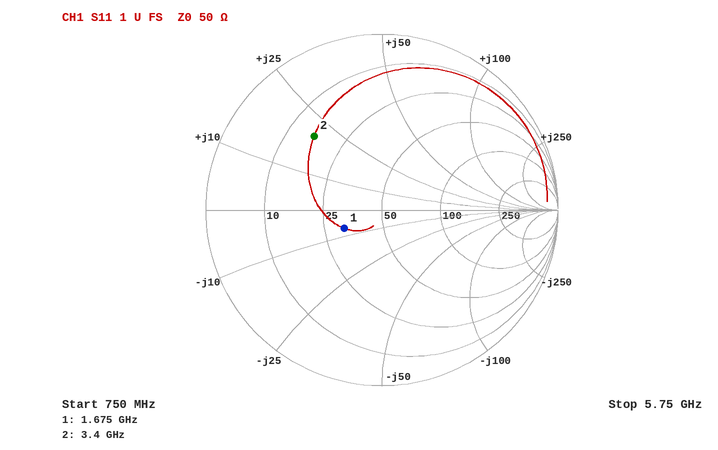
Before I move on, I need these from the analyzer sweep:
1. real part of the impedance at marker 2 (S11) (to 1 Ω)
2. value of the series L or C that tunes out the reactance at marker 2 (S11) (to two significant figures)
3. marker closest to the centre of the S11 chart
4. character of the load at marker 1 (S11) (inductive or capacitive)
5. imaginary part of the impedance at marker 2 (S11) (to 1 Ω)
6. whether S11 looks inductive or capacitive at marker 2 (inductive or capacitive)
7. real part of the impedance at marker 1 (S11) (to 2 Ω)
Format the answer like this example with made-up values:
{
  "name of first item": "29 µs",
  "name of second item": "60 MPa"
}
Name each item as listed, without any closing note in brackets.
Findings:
{
  "real part of the impedance at marker 2 (S11)": "16 Ω",
  "value of the series L or C that tunes out the reactance at marker 2 (S11)": "2.3 pF",
  "marker closest to the centre of the S11 chart": "marker 1",
  "character of the load at marker 1 (S11)": "capacitive",
  "imaginary part of the impedance at marker 2 (S11)": "+20 Ω",
  "whether S11 looks inductive or capacitive at marker 2": "inductive",
  "real part of the impedance at marker 1 (S11)": "32 Ω"
}
